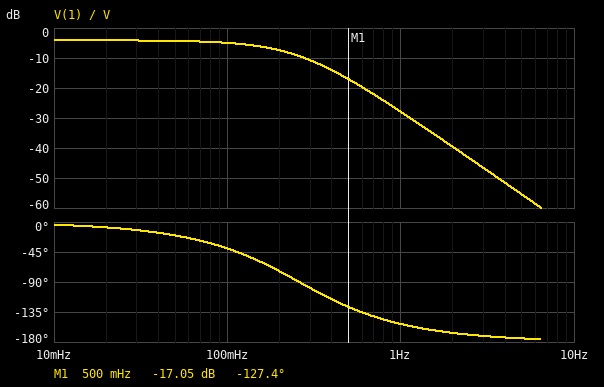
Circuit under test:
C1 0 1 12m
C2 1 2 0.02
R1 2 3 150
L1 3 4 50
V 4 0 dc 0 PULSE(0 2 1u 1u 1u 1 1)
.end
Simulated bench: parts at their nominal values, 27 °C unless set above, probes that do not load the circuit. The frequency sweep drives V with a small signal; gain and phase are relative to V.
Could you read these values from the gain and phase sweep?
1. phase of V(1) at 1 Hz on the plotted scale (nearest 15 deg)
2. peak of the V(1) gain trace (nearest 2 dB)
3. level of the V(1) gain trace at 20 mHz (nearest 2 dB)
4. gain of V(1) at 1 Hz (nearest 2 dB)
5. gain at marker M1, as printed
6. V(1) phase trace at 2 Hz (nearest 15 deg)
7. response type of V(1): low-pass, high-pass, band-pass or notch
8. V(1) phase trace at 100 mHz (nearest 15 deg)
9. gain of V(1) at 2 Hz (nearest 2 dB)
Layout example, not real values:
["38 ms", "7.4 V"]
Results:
["-150 deg", "-4 dB", "-4 dB", "-28 dB", "-17.05 dB", "-165 deg", "low-pass", "-45 deg", "-40 dB"]
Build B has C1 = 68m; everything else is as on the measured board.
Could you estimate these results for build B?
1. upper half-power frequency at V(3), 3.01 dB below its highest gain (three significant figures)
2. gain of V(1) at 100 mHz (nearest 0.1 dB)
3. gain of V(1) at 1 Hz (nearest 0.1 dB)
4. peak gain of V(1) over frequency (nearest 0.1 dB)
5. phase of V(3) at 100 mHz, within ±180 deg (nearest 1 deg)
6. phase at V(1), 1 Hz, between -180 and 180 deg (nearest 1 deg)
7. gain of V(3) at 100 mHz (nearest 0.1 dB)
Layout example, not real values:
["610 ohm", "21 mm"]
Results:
["469 mHz", "-17.0 dB", "-43.2 dB", "-12.9 dB", "-9 deg", "-154 deg", "0.8 dB"]
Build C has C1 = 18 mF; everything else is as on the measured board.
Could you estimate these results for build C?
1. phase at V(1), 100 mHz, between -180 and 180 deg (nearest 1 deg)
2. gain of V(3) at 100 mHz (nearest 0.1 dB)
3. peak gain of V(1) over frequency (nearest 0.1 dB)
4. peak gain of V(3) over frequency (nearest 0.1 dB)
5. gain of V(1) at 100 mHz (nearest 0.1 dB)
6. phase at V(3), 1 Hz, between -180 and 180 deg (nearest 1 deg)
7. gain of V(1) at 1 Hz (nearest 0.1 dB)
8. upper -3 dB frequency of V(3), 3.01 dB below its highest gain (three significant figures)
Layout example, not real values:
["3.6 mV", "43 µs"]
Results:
["-48 deg", "0.9 dB", "-5.6 dB", "1.2 dB", "-7.2 dB", "-70 deg", "-31.5 dB", "482 mHz"]
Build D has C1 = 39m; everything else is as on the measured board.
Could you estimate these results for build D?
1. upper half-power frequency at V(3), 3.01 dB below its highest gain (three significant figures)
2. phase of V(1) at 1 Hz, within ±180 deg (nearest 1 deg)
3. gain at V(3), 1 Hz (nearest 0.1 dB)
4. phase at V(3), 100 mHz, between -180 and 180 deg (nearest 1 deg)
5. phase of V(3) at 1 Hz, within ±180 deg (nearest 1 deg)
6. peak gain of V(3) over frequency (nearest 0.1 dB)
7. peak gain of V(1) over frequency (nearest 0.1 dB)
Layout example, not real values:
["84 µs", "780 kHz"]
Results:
["471 mHz", "-154 deg", "-7.0 dB", "-8 deg", "-68 deg", "0.9 dB", "-9.4 dB"]
